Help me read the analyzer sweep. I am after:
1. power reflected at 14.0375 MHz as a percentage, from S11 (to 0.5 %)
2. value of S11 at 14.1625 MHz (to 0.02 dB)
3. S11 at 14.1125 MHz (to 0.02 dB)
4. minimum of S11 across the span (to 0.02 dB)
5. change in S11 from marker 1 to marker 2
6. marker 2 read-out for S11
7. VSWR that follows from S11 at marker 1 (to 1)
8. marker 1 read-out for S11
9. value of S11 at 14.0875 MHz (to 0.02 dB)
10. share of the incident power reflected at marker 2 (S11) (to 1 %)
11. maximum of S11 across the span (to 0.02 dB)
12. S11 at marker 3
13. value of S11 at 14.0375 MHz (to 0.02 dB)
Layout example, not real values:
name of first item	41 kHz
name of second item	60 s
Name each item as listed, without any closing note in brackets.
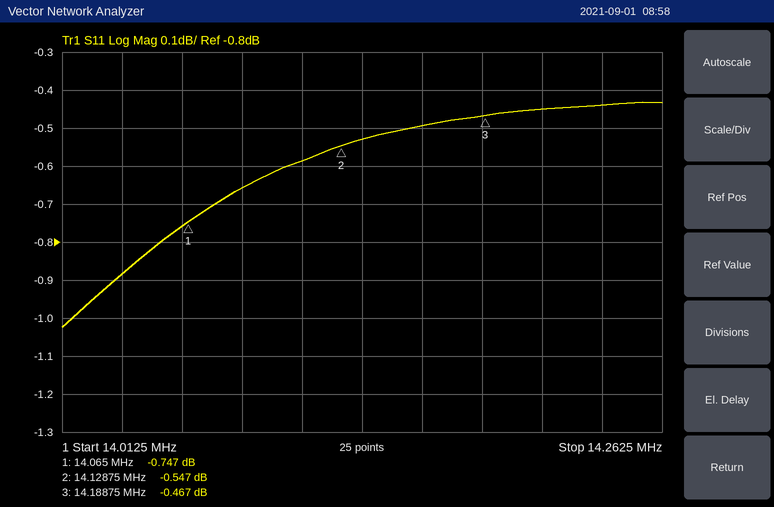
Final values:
power reflected at 14.0375 MHz as a percentage, from S11	81.5 %
value of S11 at 14.1625 MHz	-0.50 dB
S11 at 14.1125 MHz	-0.58 dB
minimum of S11 across the span	-1.02 dB
change in S11 from marker 1 to marker 2	0.200 dB
marker 2 read-out for S11	-0.547 dB
VSWR that follows from S11 at marker 1	23
marker 1 read-out for S11	-0.747 dB
value of S11 at 14.0875 MHz	-0.66 dB
share of the incident power reflected at marker 2 (S11)	88 %
maximum of S11 across the span	-0.44 dB
S11 at marker 3	-0.467 dB
value of S11 at 14.0375 MHz	-0.88 dB
